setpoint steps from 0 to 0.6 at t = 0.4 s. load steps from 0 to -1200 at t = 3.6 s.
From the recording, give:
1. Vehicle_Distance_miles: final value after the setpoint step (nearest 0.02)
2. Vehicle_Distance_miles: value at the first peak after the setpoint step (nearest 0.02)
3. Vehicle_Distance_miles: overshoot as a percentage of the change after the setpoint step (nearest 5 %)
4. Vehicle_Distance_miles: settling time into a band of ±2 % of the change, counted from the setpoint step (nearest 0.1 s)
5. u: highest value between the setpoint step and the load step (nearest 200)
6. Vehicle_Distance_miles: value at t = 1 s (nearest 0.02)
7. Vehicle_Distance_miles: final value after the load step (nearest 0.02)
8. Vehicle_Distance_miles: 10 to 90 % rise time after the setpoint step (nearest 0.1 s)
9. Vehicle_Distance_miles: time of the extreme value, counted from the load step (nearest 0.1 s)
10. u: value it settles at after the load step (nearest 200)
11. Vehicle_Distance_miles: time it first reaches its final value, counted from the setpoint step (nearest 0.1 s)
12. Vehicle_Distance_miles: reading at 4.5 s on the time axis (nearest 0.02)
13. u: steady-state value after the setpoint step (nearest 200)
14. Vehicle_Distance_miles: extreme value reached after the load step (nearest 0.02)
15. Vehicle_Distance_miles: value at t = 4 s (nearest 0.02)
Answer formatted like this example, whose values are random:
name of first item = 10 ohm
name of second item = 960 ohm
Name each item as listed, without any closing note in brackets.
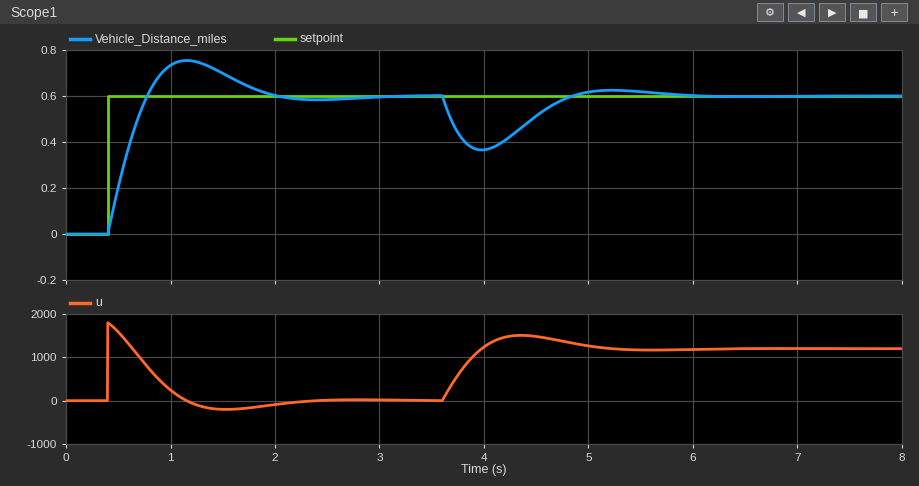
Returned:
Vehicle_Distance_miles: final value after the setpoint step = 0.60
Vehicle_Distance_miles: value at the first peak after the setpoint step = 0.76
Vehicle_Distance_miles: overshoot as a percentage of the change after the setpoint step = 25 %
Vehicle_Distance_miles: settling time into a band of ±2 % of the change, counted from the setpoint step = 2.3 s
u: highest value between the setpoint step and the load step = 1800
Vehicle_Distance_miles: value at t = 1 s = 0.74
Vehicle_Distance_miles: final value after the load step = 0.60
Vehicle_Distance_miles: 10 to 90 % rise time after the setpoint step = 0.3 s
Vehicle_Distance_miles: time of the extreme value, counted from the load step = 0.4 s
u: value it settles at after the load step = 1200
Vehicle_Distance_miles: time it first reaches its final value, counted from the setpoint step = 0.4 s
Vehicle_Distance_miles: reading at 4.5 s on the time axis = 0.52
u: steady-state value after the setpoint step = 0
Vehicle_Distance_miles: extreme value reached after the load step = 0.36
Vehicle_Distance_miles: value at t = 4 s = 0.36
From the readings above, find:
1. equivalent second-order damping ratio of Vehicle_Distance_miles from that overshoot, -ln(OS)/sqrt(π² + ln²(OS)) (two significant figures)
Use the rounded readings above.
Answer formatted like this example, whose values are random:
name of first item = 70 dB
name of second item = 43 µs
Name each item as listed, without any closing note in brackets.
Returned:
equivalent second-order damping ratio of Vehicle_Distance_miles from that overshoot, -ln(OS)/sqrt(π² + ln²(OS)) = 0.40
